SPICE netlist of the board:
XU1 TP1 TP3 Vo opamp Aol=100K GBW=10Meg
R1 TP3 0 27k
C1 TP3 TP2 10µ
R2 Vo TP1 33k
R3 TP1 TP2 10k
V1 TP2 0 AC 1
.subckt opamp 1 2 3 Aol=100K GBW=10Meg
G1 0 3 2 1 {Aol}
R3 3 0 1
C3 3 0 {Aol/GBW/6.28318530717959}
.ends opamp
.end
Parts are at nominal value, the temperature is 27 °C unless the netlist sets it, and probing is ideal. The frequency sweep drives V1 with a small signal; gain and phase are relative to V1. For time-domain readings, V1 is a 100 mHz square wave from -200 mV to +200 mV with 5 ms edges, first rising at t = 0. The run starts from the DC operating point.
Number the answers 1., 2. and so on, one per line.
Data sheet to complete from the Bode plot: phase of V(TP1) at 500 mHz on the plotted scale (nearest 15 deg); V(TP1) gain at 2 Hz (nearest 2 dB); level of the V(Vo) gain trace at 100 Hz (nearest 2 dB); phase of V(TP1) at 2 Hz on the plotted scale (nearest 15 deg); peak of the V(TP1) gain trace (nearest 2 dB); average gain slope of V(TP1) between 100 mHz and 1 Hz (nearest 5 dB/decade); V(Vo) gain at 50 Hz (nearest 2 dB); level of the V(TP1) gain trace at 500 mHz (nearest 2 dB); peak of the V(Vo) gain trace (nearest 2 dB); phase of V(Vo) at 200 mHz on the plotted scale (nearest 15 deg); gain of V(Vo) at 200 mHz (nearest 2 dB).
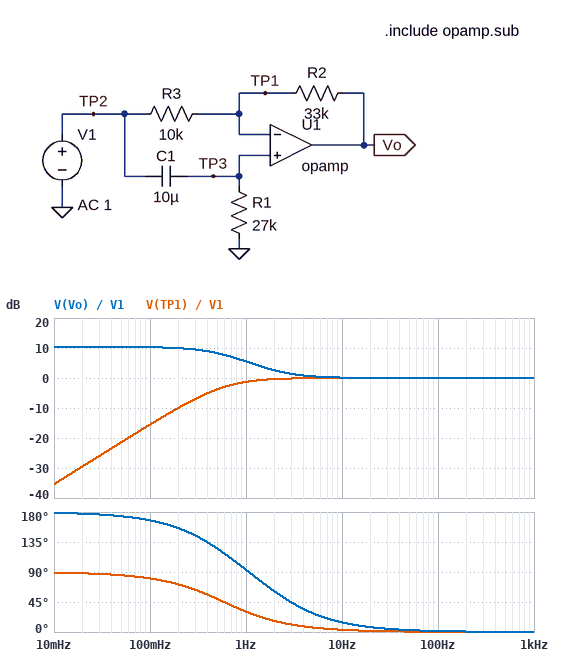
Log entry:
1. 45 deg
2. 0 dB
3. 0 dB
4. 15 deg
5. 0 dB
6. 15 dB/decade
7. 0 dB
8. -4 dB
9. 10 dB
10. 150 deg
11. 10 dB
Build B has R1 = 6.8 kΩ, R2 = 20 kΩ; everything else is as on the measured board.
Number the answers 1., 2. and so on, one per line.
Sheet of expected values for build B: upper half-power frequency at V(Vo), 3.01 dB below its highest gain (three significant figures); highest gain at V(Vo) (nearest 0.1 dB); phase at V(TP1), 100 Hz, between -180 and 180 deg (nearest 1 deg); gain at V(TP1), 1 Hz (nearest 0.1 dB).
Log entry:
1. 3.31 Hz
2. 6.0 dB
3. 1 deg
4. -8.1 dB
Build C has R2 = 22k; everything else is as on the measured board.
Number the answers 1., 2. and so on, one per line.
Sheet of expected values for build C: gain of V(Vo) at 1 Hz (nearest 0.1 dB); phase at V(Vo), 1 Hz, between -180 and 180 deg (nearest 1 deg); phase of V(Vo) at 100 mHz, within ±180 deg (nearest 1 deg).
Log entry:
1. 3.0 dB
2. 83 deg
3. 166 deg
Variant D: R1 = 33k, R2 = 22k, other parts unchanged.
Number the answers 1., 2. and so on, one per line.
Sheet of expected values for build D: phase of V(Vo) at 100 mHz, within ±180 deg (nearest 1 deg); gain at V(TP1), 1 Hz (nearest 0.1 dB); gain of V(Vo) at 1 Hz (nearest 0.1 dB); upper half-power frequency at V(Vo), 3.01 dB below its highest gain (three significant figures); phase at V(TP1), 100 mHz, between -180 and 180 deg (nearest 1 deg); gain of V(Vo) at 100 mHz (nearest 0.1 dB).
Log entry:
1. 163 deg
2. -0.9 dB
3. 2.4 dB
4. 630 mHz
5. 78 deg
6. 6.7 dB
